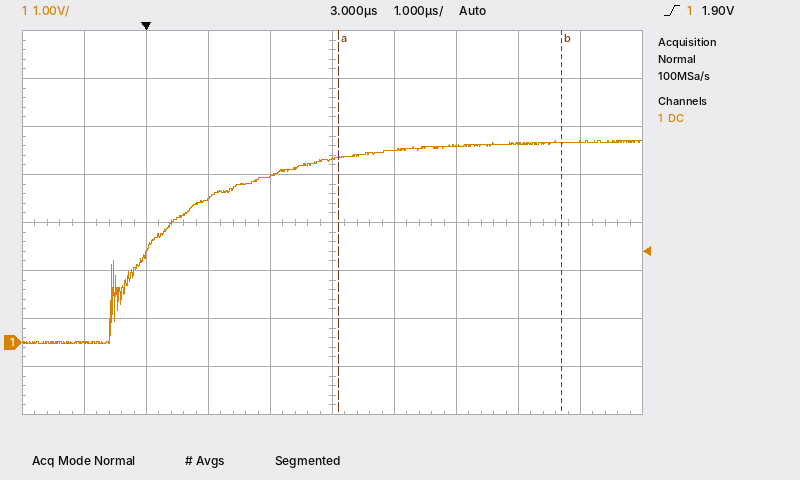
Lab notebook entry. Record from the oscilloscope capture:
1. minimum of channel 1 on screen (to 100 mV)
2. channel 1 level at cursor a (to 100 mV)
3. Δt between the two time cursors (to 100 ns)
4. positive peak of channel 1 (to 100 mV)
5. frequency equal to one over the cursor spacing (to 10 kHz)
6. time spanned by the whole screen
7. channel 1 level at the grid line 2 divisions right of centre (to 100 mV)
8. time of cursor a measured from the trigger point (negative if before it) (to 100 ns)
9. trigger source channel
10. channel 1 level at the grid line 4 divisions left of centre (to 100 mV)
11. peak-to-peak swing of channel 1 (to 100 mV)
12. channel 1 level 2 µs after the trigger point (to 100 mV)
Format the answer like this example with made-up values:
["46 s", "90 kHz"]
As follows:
["0.0 V", "3.9 V", "3.6 µs", "4.2 V", "280 kHz", "10 µs", "4.1 V", "+3.1 µs", "channel 1", "0.0 V", "4.2 V", "3.5 V"]
